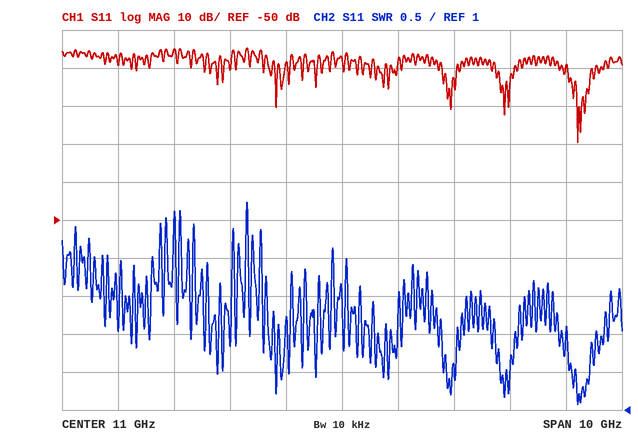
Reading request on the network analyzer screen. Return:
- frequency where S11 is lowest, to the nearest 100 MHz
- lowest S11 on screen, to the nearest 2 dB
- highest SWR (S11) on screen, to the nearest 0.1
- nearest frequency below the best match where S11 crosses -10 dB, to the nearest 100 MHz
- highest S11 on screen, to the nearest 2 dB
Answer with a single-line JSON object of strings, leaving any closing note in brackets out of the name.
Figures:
{"frequency where S11 is lowest, to the nearest 100 MHz": "15.2 GHz", "lowest S11 on screen, to the nearest 2 dB": "-30 dB", "highest SWR (S11) on screen, to the nearest 0.1": "3.7", "nearest frequency below the best match where S11 crosses -10 dB, to the nearest 100 MHz": "15.0 GHz", "highest S11 on screen, to the nearest 2 dB": "-4 dB"}
